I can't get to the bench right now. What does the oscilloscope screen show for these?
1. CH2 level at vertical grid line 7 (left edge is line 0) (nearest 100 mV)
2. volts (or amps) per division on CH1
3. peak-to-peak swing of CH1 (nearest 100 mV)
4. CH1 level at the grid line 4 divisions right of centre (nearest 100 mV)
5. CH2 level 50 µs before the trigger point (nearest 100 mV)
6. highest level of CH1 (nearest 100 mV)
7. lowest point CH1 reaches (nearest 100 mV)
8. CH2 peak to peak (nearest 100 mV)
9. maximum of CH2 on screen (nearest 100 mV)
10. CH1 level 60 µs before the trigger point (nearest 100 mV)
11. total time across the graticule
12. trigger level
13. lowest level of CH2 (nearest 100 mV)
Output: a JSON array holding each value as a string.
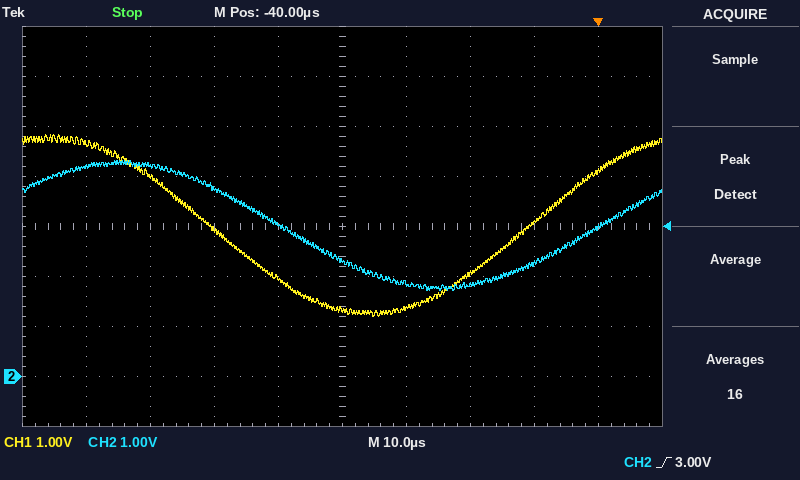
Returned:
["1.8 V", "1 V", "3.6 V", "4.1 V", "3.0 V", "4.8 V", "1.2 V", "2.6 V", "4.3 V", "2.9 V", "100 µs", "3.00 V", "1.7 V"]
